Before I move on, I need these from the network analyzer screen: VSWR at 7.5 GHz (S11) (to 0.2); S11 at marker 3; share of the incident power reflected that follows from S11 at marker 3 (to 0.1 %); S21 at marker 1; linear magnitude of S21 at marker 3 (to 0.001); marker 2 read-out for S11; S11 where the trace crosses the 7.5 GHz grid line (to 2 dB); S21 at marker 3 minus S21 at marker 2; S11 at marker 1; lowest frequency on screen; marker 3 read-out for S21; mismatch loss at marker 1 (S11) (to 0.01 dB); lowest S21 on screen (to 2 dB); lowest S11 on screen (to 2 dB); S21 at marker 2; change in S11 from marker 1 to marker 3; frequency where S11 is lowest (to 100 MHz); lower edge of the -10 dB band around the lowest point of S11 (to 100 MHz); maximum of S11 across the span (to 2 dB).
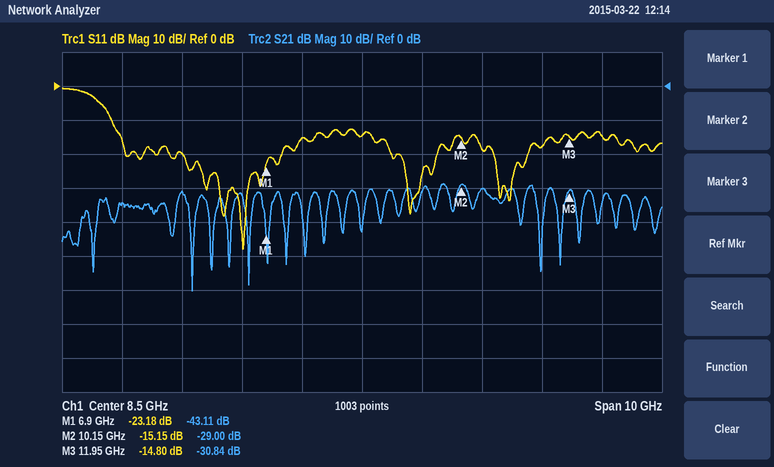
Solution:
1.4
-14.80 dB
3.3 %
-43.11 dB
0.029
-15.15 dB
-16 dB
-1.84 dB
-23.18 dB
3.5 GHz
-30.84 dB
0.02 dB
-60 dB
-48 dB
-29.00 dB
8.38 dB
6.5 GHz
4.3 GHz
0 dB
